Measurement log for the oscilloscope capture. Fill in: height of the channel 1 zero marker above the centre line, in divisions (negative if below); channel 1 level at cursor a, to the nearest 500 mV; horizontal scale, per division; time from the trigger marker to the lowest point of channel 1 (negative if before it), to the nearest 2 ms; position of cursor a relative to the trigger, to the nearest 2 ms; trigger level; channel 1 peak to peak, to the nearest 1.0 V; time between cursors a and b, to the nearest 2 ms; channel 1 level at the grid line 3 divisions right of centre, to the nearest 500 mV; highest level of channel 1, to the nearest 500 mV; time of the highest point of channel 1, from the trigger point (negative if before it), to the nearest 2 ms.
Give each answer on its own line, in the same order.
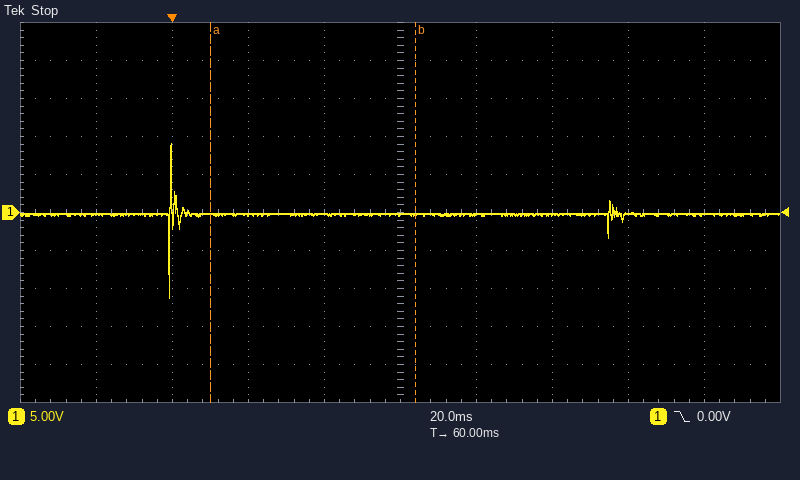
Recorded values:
0.0 div
0.0 V
20 ms
0 ms
+10 ms
0.00 V
20.0 V
54 ms
0.0 V
9.0 V
0 ms
